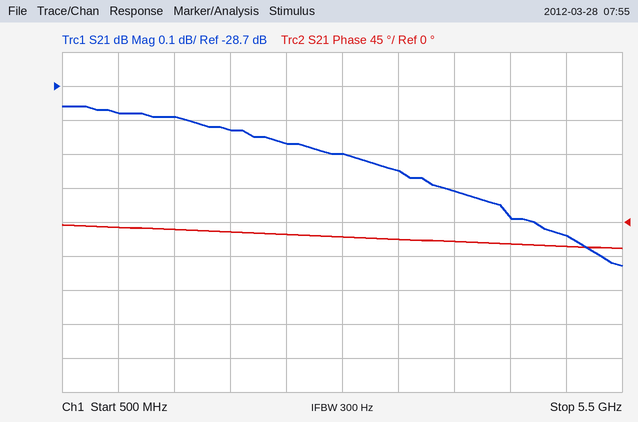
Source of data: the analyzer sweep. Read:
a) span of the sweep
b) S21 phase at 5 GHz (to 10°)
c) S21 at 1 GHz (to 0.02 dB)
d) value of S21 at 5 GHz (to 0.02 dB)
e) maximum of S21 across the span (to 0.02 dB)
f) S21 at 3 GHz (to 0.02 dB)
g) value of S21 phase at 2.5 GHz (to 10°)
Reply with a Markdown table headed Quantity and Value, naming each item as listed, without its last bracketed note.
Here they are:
| Quantity | Value |
|---|---|
| span of the sweep | 5 GHz |
| S21 phase at 5 GHz | -30° |
| S21 at 1 GHz | -28.78 dB |
| value of S21 at 5 GHz | -29.14 dB |
| maximum of S21 across the span | -28.76 dB |
| S21 at 3 GHz | -28.90 dB |
| value of S21 phase at 2.5 GHz | -20° |
